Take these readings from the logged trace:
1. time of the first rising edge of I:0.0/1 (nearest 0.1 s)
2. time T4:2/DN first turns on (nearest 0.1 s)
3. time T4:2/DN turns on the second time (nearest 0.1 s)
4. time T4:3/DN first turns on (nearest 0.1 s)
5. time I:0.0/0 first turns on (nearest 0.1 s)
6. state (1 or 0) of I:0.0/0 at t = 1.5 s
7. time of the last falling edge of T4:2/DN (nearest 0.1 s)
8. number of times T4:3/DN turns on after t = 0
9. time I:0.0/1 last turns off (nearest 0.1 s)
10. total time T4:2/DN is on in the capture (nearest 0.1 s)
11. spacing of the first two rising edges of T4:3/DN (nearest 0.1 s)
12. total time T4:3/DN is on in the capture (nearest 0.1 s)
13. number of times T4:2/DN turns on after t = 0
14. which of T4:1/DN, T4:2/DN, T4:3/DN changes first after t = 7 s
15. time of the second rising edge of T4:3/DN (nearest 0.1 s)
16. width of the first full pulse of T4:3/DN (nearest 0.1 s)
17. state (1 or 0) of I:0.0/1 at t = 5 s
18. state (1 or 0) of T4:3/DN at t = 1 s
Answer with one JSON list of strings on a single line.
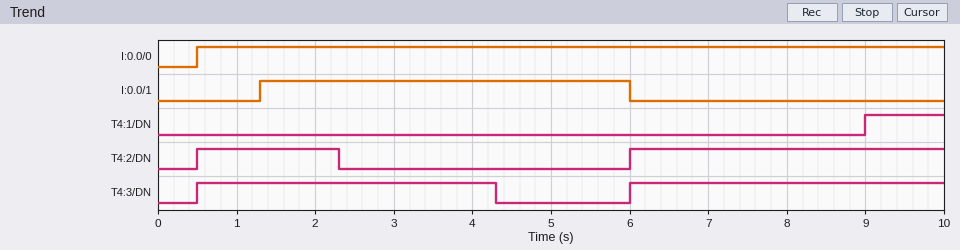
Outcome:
["1.3 s", "0.5 s", "6.0 s", "0.5 s", "0.5 s", "1", "2.3 s", "2", "6.0 s", "5.8 s", "5.5 s", "7.8 s", "2", "T4:1/DN", "6.0 s", "3.8 s", "1", "1"]
